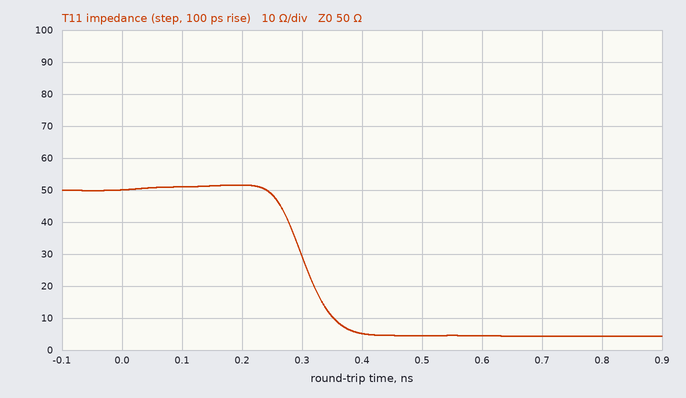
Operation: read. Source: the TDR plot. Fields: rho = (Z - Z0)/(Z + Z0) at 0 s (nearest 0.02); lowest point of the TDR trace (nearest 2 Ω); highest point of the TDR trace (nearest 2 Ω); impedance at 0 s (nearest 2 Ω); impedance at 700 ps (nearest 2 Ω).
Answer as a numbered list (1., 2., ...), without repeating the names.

1. 0.00
2. 4 Ω
3. 52 Ω
4. 50 Ω
5. 4 Ω
